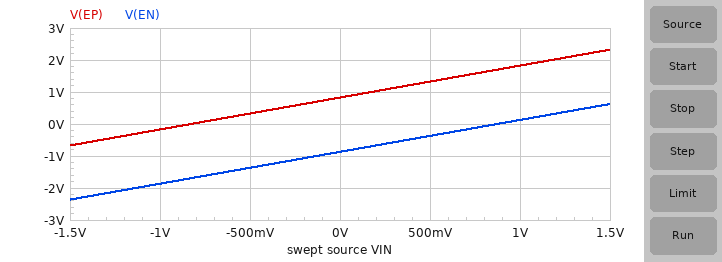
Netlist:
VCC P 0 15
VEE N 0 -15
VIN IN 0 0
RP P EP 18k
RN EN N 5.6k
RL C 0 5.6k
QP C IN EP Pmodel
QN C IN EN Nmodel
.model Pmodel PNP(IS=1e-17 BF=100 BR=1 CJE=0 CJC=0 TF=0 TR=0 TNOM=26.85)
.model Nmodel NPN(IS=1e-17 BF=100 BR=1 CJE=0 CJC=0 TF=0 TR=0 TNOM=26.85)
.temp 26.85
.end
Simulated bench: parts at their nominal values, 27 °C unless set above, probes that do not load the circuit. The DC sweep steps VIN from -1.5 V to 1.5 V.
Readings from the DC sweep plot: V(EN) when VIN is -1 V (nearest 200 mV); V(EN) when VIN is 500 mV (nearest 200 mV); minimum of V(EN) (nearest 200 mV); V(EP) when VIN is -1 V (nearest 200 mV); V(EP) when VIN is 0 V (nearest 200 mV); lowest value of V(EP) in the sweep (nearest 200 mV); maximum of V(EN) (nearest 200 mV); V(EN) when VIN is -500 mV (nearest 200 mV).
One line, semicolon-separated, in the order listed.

-1.8 V; -400 mV; -2.4 V; -200 mV; 800 mV; -600 mV; 600 mV; -1.4 V
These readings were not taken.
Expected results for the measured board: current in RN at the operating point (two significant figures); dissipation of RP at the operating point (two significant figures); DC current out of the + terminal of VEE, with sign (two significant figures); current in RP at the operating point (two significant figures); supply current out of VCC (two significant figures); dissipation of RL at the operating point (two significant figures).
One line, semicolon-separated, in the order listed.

2.5 mA; 11 mW; -2.5 mA; 790 µA; 790 µA; 130 µW
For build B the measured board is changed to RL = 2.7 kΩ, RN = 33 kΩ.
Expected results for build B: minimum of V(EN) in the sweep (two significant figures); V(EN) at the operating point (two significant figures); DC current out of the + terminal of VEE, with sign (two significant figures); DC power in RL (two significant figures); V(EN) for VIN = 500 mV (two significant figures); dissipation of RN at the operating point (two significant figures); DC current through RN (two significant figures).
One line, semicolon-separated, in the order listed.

-2.3 V; -810 mV; -430 µA; 220 µW; -310 mV; 6.1 mW; 430 µA
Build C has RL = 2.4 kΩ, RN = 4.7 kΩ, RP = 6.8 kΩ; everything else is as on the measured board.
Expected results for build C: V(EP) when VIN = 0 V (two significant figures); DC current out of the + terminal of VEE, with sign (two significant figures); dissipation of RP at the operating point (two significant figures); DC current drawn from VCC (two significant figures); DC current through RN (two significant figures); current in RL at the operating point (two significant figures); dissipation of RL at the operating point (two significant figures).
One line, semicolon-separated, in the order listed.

850 mV; -3.0 mA; 29 mW; 2.1 mA; 3.0 mA; 340 µA; 280 µW
